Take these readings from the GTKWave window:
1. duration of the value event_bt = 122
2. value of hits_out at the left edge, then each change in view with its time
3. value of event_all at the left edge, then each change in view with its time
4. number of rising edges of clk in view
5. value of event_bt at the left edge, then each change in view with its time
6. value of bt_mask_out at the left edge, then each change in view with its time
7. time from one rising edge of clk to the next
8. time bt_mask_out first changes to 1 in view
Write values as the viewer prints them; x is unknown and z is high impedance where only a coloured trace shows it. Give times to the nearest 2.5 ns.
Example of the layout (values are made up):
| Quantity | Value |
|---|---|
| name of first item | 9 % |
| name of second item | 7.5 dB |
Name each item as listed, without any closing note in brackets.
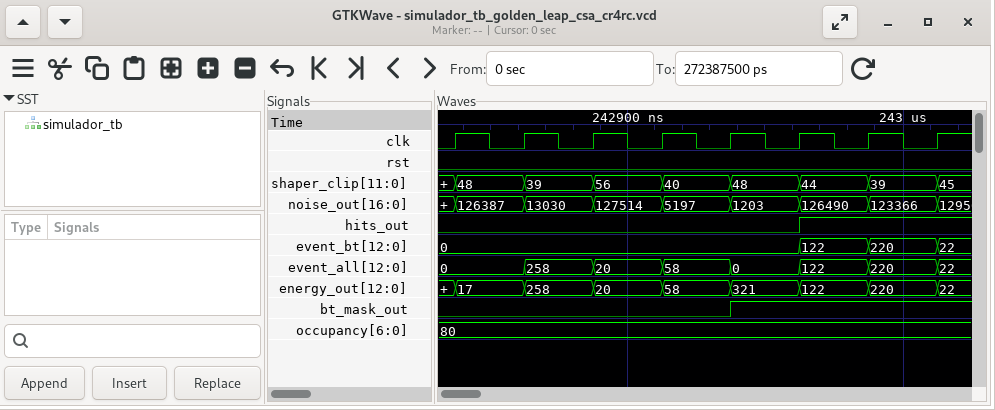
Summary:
| Quantity | Value |
|---|---|
| duration of the value event_bt = 122 | 25 ns |
| value of hits_out at the left edge, then each change in view with its time | 0, 1 at 242962.5 ns |
| value of event_all at the left edge, then each change in view with its time | 0, 258 at 242862.5 ns, 20 at 242887.5 ns, 58 at 242912.5 ns, 0 at 242937.5 ns, 122 at 242962.5 ns, 220 at 242987.5 ns, 22 at 243012.5 ns |
| number of rising edges of clk in view | 8 |
| value of event_bt at the left edge, then each change in view with its time | 0, 122 at 242962.5 ns, 220 at 242987.5 ns, 22 at 243012.5 ns |
| value of bt_mask_out at the left edge, then each change in view with its time | 0, 1 at 242937.5 ns |
| time from one rising edge of clk to the next | 25 ns |
| time bt_mask_out first changes to 1 in view | 242937.5 ns |
